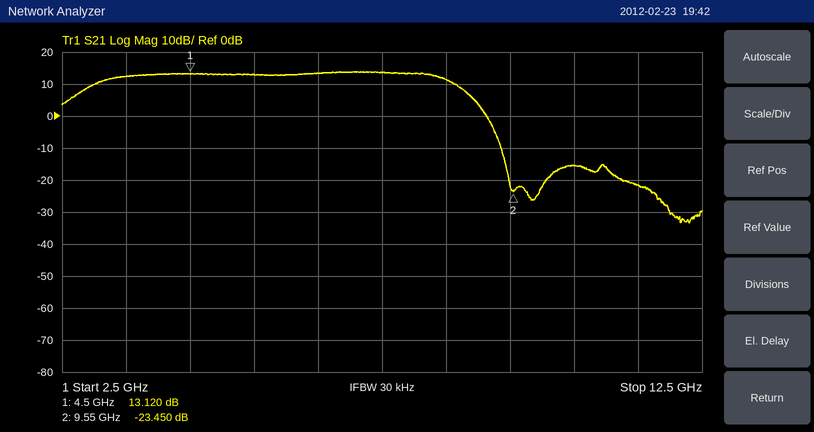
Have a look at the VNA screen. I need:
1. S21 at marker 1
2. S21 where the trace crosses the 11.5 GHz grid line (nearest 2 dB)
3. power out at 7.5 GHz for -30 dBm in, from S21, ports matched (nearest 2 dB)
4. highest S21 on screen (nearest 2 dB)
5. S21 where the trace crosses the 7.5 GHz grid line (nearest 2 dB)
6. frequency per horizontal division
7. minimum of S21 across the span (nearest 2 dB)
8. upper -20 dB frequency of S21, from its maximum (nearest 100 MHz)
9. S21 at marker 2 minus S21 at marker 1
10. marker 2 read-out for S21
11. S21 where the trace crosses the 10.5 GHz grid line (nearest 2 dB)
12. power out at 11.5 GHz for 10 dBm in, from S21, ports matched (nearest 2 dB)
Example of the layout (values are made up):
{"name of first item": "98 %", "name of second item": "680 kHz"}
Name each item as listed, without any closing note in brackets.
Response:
{"S21 at marker 1": "13.120 dB", "S21 where the trace crosses the 11.5 GHz grid line": "-22 dB", "power out at 7.5 GHz for -30 dBm in, from S21, ports matched": "-16 dBm", "highest S21 on screen": "14 dB", "S21 where the trace crosses the 7.5 GHz grid line": "14 dB", "frequency per horizontal division": "1 GHz", "minimum of S21 across the span": "-34 dB", "upper -20 dB frequency of S21, from its maximum": "9.3 GHz", "S21 at marker 2 minus S21 at marker 1": "-36.570 dB", "marker 2 read-out for S21": "-23.450 dB", "S21 where the trace crosses the 10.5 GHz grid line": "-16 dB", "power out at 11.5 GHz for 10 dBm in, from S21, ports matched": "-12 dBm"}
